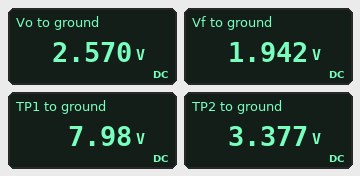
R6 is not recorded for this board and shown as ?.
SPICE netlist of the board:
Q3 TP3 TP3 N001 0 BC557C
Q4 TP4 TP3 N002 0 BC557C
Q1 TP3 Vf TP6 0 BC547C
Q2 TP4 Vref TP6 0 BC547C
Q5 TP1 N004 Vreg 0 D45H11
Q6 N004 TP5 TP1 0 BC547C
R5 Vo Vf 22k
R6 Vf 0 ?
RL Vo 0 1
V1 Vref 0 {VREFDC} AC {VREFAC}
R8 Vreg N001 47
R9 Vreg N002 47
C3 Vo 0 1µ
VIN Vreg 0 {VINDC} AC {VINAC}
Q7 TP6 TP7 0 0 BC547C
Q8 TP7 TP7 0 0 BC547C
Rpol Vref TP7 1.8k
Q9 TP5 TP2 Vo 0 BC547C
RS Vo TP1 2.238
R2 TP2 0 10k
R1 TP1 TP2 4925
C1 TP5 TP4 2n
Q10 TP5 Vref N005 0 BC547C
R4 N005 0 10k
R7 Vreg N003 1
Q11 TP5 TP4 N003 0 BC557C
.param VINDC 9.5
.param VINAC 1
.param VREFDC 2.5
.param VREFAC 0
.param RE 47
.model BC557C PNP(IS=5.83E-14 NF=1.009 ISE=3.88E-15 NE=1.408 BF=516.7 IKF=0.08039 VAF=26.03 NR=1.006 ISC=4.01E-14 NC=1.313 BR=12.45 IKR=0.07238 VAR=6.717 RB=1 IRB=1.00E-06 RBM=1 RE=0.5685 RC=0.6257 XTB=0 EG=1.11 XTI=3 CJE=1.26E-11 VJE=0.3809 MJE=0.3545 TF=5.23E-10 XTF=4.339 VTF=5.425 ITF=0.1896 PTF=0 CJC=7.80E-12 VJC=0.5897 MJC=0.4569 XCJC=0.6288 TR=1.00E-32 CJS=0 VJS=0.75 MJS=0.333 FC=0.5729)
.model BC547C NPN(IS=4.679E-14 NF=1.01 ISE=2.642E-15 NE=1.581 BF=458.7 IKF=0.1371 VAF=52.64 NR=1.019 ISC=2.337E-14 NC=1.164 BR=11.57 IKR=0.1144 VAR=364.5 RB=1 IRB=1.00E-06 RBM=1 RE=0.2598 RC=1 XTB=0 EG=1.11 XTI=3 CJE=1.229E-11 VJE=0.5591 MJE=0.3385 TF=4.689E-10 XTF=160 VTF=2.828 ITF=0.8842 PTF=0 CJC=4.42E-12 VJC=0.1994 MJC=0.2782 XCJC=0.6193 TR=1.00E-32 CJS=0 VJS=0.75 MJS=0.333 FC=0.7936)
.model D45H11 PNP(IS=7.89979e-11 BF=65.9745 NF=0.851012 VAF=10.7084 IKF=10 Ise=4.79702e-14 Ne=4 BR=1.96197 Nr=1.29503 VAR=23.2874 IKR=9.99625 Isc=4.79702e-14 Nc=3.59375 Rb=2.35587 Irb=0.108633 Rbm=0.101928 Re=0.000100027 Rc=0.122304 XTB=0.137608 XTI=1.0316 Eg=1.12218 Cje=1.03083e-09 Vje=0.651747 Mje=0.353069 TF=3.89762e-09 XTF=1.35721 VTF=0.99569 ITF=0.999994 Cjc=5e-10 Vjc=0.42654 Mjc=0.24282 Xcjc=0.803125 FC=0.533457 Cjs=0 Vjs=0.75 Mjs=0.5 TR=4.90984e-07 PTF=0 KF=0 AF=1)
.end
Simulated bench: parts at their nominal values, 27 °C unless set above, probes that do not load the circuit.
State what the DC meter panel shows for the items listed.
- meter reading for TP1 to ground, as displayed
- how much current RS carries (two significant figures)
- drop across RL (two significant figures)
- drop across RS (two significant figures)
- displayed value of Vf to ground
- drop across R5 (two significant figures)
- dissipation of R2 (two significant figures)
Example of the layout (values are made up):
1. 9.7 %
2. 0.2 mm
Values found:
1. 7.98 V
2. 2.4 A
3. 2.6 V
4. 5.4 V
5. 1.942 V
6. 630 mV
7. 1.1 mW
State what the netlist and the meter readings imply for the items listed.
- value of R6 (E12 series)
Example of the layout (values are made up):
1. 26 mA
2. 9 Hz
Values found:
1. 68 kΩ
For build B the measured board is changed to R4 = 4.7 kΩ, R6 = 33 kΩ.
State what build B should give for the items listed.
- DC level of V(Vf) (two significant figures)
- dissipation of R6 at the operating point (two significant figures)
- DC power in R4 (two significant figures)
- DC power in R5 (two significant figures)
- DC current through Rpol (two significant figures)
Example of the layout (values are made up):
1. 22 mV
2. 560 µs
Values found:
1. 1.5 V
2. 72 µW
3. 770 µW
4. 48 µW
5. 1.0 mA
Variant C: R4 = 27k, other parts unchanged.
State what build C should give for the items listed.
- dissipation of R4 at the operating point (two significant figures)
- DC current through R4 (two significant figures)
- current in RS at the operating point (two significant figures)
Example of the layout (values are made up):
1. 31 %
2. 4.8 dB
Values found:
1. 140 µW
2. 72 µA
3. 2.4 A
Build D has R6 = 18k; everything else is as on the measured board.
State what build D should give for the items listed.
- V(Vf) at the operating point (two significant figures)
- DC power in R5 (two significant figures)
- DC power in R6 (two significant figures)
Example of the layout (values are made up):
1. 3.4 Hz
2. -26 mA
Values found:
1. 1.2 V
2. 91 µW
3. 74 µW
